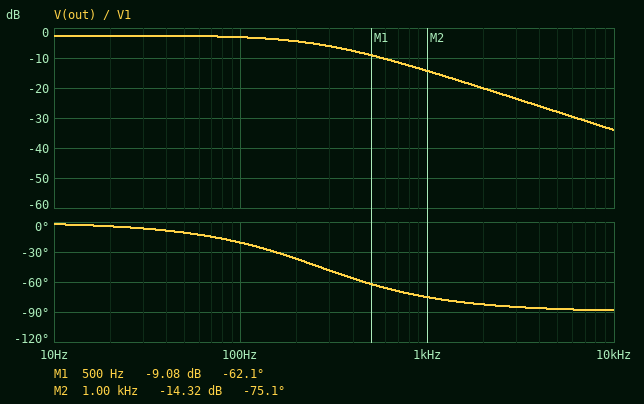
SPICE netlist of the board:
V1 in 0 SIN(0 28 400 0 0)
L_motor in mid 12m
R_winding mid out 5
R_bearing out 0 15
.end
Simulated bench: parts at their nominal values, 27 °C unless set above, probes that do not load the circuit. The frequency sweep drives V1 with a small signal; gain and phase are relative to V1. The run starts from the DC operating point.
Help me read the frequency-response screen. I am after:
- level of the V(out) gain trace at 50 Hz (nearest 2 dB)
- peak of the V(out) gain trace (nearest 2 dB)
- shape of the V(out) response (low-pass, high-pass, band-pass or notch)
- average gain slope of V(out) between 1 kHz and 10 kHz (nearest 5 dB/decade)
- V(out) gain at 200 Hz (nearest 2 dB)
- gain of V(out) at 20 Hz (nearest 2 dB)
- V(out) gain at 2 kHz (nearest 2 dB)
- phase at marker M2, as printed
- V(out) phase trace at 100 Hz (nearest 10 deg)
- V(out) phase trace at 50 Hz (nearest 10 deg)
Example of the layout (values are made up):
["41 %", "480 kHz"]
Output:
["-2 dB", "-2 dB", "low-pass", "-20 dB/decade", "-4 dB", "-2 dB", "-20 dB", "-75.1 deg", "-20 deg", "-10 deg"]
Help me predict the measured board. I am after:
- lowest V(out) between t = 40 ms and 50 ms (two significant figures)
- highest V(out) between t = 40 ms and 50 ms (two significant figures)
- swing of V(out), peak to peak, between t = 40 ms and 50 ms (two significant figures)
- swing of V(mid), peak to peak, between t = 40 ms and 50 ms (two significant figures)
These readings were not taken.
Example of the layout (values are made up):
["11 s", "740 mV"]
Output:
["-12 V", "12 V", "23 V", "31 V"]
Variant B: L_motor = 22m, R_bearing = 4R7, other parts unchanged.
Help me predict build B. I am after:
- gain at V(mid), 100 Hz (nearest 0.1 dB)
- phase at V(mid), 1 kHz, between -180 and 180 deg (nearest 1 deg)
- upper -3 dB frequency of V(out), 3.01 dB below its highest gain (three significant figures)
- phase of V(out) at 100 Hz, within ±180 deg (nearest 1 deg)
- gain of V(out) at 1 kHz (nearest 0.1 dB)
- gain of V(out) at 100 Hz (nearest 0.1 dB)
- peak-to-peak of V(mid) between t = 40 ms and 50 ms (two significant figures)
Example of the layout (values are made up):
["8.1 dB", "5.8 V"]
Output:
["-4.8 dB", "-86 deg", "70.2 Hz", "-55 deg", "-29.4 dB", "-11.1 dB", "9.7 V"]
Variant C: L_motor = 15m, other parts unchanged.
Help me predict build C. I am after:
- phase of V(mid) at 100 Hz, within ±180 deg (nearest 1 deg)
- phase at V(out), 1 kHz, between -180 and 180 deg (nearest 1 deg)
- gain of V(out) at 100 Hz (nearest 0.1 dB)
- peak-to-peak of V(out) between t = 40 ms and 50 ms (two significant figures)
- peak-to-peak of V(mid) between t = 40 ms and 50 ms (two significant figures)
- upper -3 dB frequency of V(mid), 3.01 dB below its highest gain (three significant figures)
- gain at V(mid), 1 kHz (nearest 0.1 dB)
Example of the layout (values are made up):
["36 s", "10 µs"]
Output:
["-25 deg", "-78 deg", "-3.4 dB", "20 V", "26 V", "212 Hz", "-13.7 dB"]
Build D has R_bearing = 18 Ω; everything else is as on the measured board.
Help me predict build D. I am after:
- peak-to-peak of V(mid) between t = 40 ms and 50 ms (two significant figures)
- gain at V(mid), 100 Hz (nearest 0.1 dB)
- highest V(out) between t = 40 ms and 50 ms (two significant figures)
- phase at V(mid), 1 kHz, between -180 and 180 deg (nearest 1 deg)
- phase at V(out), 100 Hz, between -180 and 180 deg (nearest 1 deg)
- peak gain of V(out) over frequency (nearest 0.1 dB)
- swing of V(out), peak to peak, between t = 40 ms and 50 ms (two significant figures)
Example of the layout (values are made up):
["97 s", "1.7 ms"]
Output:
["34 V", "-0.4 dB", "13 V", "-73 deg", "-18 deg", "-2.1 dB", "27 V"]
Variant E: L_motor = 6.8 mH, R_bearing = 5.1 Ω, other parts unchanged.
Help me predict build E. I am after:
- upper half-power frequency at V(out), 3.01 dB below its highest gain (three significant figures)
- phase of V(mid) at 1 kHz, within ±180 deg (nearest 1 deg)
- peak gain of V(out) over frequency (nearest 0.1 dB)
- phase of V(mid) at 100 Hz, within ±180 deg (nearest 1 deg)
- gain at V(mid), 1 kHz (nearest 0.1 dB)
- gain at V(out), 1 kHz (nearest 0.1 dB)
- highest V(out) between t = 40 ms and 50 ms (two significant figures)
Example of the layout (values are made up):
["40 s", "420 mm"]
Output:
["236 Hz", "-77 deg", "-5.9 dB", "-23 deg", "-12.8 dB", "-18.7 dB", "7.2 V"]
